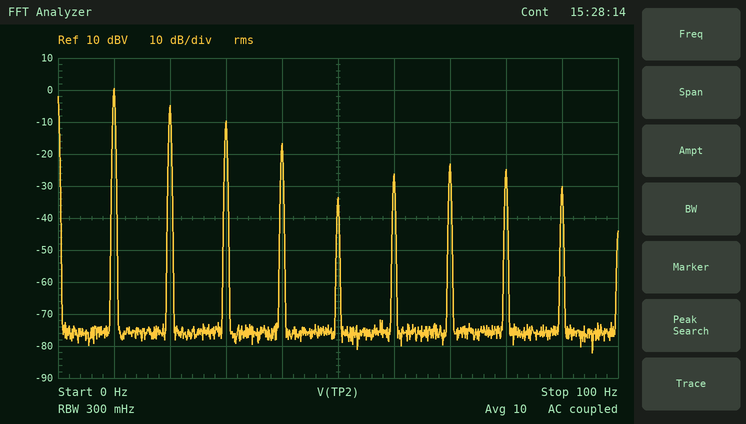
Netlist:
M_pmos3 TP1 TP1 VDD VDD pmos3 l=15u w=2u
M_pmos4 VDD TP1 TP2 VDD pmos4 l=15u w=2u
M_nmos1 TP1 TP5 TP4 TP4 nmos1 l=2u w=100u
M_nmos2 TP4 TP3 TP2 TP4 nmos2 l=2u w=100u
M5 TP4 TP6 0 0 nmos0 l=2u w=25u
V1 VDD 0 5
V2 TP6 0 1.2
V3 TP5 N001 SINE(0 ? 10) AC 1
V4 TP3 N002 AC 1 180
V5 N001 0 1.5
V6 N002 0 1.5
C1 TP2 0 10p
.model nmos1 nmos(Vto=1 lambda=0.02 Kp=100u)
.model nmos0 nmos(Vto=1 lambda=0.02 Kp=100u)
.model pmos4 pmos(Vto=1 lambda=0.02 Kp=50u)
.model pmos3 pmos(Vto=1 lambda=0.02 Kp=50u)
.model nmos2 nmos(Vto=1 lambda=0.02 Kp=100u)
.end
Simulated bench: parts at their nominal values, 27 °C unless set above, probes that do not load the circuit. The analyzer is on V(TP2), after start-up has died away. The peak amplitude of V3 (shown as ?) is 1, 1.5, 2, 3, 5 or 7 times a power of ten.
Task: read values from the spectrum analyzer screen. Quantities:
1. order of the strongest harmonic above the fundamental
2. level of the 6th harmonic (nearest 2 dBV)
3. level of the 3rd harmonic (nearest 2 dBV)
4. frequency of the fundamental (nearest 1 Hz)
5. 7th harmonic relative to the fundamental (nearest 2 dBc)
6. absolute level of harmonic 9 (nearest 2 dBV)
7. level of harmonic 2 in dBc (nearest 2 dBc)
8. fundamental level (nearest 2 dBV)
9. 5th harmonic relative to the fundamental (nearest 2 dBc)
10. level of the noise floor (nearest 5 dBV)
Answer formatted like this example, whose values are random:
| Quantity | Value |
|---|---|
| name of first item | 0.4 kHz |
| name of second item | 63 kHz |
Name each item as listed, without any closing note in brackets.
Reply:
| Quantity | Value |
|---|---|
| order of the strongest harmonic above the fundamental | 2 |
| level of the 6th harmonic | -26 dBV |
| level of the 3rd harmonic | -10 dBV |
| frequency of the fundamental | 10 Hz |
| 7th harmonic relative to the fundamental | -24 dBc |
| absolute level of harmonic 9 | -30 dBV |
| level of harmonic 2 in dBc | -6 dBc |
| fundamental level | 0 dBV |
| 5th harmonic relative to the fundamental | -34 dBc |
| level of the noise floor | -75 dBV |
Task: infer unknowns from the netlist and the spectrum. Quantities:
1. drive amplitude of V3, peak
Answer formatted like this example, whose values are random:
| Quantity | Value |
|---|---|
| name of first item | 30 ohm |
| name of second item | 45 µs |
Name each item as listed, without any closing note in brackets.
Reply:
| Quantity | Value |
|---|---|
| drive amplitude of V3, peak | 15 mV |
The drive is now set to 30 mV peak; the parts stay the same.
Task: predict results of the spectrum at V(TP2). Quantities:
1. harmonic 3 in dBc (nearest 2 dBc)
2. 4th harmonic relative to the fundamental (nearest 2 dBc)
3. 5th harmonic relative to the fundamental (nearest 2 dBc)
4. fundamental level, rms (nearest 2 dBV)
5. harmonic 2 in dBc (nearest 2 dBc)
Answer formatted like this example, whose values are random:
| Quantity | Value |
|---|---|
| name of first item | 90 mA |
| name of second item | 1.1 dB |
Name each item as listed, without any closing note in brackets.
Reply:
| Quantity | Value |
|---|---|
| harmonic 3 in dBc | -18 dBc |
| 4th harmonic relative to the fundamental | -14 dBc |
| 5th harmonic relative to the fundamental | -24 dBc |
| fundamental level, rms | 4 dBV |
| harmonic 2 in dBc | -12 dBc |
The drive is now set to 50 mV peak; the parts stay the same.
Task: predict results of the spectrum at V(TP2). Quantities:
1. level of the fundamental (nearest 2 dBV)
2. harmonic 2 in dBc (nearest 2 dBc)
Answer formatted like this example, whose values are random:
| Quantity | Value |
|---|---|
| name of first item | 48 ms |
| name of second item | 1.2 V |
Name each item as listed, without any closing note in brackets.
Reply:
| Quantity | Value |
|---|---|
| level of the fundamental | 6 dBV |
| harmonic 2 in dBc | -18 dBc |
